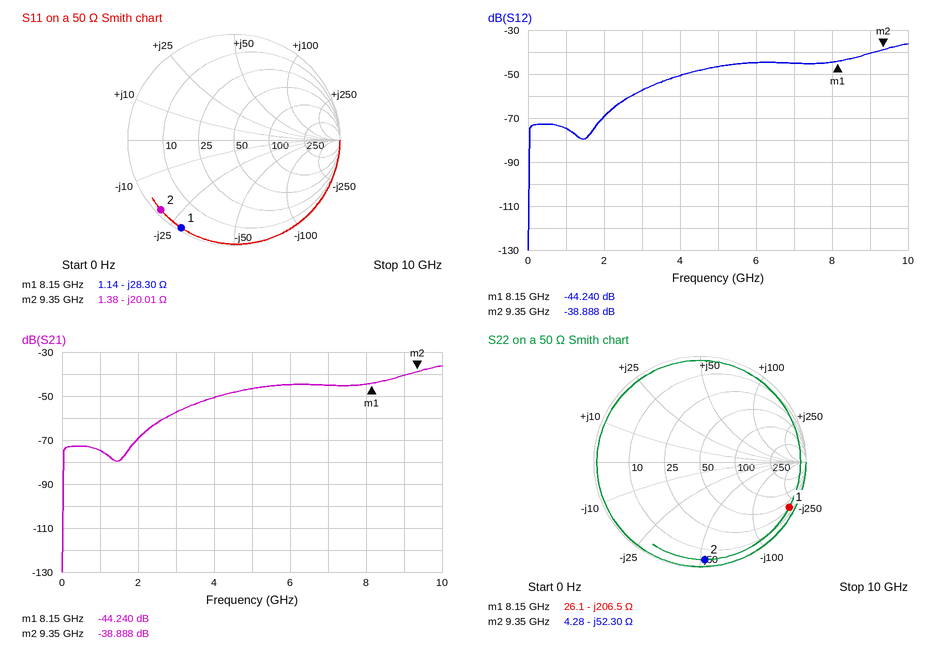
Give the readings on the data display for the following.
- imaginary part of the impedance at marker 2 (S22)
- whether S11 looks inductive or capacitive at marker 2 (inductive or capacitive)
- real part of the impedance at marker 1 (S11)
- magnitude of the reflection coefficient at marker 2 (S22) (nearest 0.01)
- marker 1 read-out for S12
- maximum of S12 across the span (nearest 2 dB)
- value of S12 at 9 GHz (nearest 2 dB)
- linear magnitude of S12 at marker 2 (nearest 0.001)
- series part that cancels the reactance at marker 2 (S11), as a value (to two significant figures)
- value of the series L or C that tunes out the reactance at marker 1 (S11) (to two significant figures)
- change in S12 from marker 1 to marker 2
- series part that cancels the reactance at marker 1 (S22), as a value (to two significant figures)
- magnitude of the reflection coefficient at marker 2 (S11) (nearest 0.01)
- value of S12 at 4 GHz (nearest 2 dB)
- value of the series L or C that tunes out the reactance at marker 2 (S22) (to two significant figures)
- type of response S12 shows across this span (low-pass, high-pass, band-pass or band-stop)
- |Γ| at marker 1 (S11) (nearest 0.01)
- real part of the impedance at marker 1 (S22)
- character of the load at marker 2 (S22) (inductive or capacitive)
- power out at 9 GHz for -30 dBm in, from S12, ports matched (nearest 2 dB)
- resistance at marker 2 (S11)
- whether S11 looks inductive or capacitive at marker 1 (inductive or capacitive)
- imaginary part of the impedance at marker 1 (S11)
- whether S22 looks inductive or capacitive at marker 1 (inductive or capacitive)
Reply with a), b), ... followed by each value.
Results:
a) -52.30 Ω
b) capacitive
c) 1.14 Ω
d) 0.92
e) -44.240 dB
f) -36 dB
g) -40 dB
h) 0.011
i) 340 pH
j) 550 pH
k) 5.352 dB
l) 4.0 nH
m) 0.95
n) -50 dB
o) 890 pH
p) high-pass
q) 0.97
r) 26.1 Ω
s) capacitive
t) -70 dBm
u) 1.38 Ω
v) capacitive
w) -28.30 Ω
x) capacitive
